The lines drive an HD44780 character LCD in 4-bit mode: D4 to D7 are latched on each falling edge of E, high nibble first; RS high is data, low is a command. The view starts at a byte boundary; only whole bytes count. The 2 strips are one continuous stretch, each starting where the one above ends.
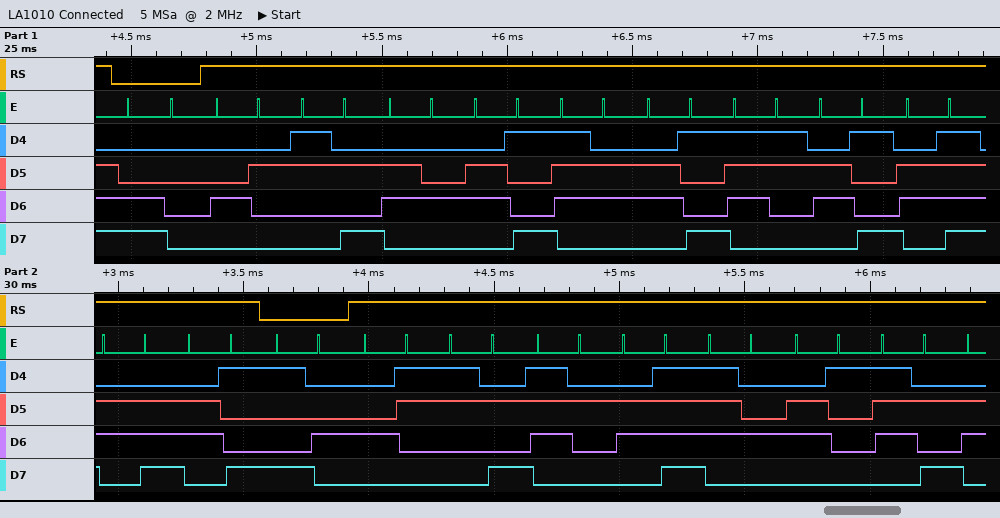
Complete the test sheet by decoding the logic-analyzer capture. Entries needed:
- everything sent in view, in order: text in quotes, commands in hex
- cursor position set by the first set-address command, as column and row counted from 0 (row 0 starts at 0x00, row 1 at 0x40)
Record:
0xC0 "B:divisioni" 0x94 "C:rotaz"
column 0, row 1
